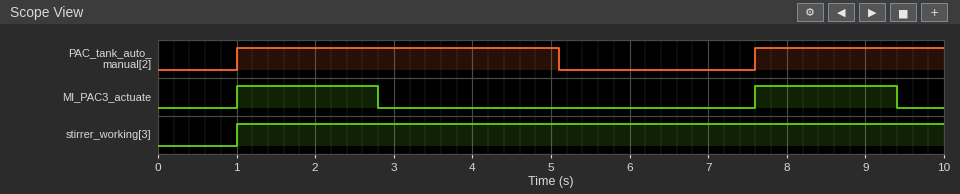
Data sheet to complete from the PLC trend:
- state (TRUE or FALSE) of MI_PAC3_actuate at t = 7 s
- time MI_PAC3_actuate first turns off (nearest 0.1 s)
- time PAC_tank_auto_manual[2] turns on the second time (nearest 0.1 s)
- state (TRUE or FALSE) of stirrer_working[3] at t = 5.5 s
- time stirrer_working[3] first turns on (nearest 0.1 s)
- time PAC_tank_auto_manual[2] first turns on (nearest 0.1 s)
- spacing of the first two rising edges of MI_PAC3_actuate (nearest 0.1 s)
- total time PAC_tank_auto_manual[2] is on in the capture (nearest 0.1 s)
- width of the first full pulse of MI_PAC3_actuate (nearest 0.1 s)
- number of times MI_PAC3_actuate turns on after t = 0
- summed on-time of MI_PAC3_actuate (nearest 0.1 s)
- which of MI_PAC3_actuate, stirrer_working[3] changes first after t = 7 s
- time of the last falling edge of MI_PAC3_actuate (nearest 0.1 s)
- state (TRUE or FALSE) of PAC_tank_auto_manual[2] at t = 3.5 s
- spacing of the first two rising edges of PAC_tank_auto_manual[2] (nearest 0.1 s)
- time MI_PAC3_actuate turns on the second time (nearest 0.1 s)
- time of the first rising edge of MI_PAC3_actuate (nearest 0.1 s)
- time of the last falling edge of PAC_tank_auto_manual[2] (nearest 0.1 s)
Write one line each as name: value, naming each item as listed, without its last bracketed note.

state (TRUE or FALSE) of MI_PAC3_actuate at t = 7 s: FALSE
time MI_PAC3_actuate first turns off: 2.8 s
time PAC_tank_auto_manual[2] turns on the second time: 7.6 s
state (TRUE or FALSE) of stirrer_working[3] at t = 5.5 s: TRUE
time stirrer_working[3] first turns on: 1.0 s
time PAC_tank_auto_manual[2] first turns on: 1.0 s
spacing of the first two rising edges of MI_PAC3_actuate: 6.6 s
total time PAC_tank_auto_manual[2] is on in the capture: 6.5 s
width of the first full pulse of MI_PAC3_actuate: 1.8 s
number of times MI_PAC3_actuate turns on after t = 0: 2
summed on-time of MI_PAC3_actuate: 3.6 s
which of MI_PAC3_actuate, stirrer_working[3] changes first after t = 7 s: MI_PAC3_actuate
time of the last falling edge of MI_PAC3_actuate: 9.4 s
state (TRUE or FALSE) of PAC_tank_auto_manual[2] at t = 3.5 s: TRUE
spacing of the first two rising edges of PAC_tank_auto_manual[2]: 6.6 s
time MI_PAC3_actuate turns on the second time: 7.6 s
time of the first rising edge of MI_PAC3_actuate: 1.0 s
time of the last falling edge of PAC_tank_auto_manual[2]: 5.1 s
